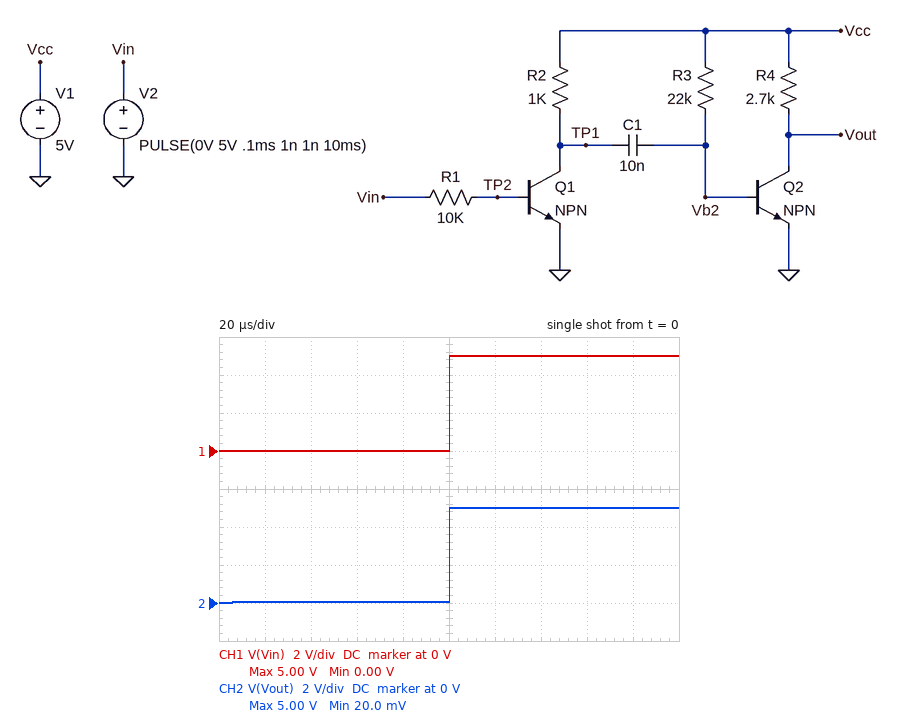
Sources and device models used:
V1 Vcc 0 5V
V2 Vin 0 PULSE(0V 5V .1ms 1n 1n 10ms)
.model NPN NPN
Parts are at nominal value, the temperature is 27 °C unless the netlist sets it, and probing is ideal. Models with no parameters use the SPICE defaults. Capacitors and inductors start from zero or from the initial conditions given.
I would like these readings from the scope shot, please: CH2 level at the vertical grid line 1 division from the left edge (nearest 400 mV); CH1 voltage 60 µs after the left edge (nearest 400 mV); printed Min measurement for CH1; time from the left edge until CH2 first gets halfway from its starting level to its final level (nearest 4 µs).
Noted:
0 V
0 V
0.00 V
100 µs
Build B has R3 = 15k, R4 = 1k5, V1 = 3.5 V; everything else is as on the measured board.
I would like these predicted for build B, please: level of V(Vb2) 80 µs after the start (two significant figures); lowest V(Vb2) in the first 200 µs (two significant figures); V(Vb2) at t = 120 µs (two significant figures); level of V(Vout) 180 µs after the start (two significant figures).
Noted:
800 mV
-2.6 V
-1.9 V
3.5 V
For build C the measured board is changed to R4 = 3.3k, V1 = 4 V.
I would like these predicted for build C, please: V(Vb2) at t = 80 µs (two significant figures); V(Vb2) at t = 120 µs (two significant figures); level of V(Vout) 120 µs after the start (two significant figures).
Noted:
780 mV
-2.5 V
4.0 V
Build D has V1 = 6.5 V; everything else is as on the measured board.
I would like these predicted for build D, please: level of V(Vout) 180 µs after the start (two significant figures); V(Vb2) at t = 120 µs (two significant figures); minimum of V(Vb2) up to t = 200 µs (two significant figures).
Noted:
6.5 V
-4.6 V
-5.6 V
